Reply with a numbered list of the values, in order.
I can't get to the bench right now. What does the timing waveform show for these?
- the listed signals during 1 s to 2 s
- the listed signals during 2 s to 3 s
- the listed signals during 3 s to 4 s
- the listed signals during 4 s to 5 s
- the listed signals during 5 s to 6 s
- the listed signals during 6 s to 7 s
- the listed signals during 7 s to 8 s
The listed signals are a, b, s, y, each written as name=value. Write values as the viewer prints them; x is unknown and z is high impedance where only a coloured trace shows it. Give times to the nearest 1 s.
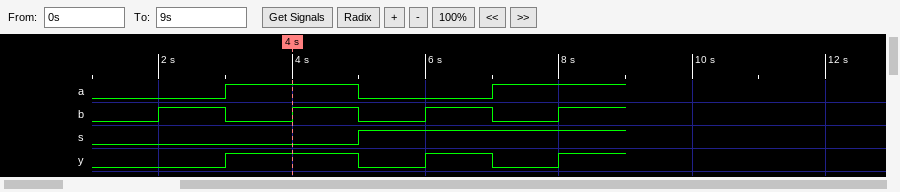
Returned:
1. a=0, b=0, s=0, y=0
2. a=0, b=1, s=0, y=0
3. a=1, b=0, s=0, y=1
4. a=1, b=1, s=0, y=1
5. a=0, b=0, s=1, y=0
6. a=0, b=1, s=1, y=1
7. a=1, b=0, s=1, y=0
